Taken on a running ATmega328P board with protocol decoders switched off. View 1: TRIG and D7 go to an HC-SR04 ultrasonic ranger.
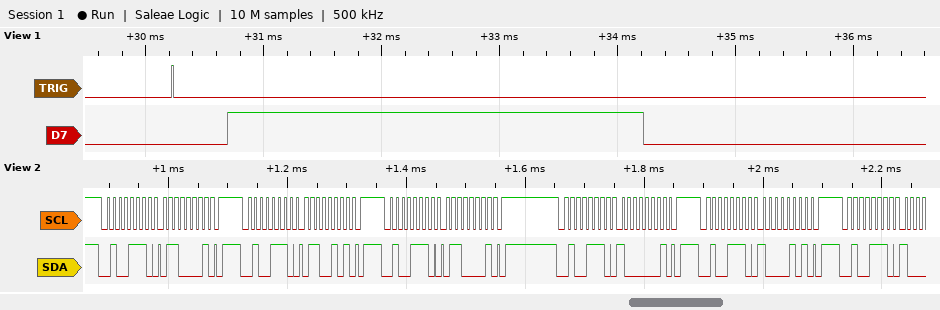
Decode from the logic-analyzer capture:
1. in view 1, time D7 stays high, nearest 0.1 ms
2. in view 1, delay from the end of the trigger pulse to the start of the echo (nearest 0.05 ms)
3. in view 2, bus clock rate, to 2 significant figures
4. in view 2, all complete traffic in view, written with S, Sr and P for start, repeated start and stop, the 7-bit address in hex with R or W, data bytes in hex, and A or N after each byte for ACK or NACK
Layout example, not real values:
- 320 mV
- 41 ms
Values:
- 3.5 ms
- 0.45 ms
- 100 kHz
- S 27W A 61 A P S 27W A 65 A P S 27W A 61 A P S 27W A 81 A P S 27W A 85 A P S 27W A
